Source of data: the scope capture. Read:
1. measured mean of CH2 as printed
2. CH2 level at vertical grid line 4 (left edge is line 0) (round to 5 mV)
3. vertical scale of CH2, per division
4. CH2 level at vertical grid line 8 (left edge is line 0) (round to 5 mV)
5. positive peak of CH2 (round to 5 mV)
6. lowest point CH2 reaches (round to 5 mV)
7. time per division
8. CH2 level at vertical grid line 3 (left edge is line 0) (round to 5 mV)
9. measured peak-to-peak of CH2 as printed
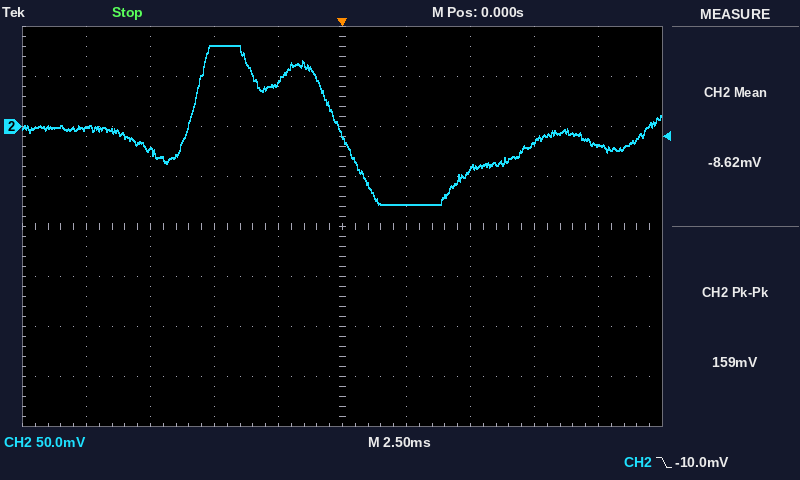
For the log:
-8.62 mV
45 mV
50 mV
-15 mV
80 mV
-80 mV
2.5 ms
80 mV
159 mV
